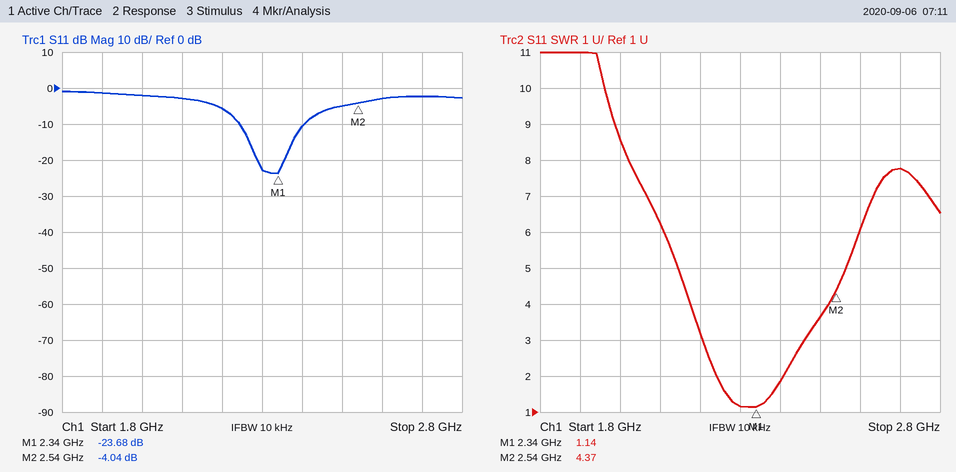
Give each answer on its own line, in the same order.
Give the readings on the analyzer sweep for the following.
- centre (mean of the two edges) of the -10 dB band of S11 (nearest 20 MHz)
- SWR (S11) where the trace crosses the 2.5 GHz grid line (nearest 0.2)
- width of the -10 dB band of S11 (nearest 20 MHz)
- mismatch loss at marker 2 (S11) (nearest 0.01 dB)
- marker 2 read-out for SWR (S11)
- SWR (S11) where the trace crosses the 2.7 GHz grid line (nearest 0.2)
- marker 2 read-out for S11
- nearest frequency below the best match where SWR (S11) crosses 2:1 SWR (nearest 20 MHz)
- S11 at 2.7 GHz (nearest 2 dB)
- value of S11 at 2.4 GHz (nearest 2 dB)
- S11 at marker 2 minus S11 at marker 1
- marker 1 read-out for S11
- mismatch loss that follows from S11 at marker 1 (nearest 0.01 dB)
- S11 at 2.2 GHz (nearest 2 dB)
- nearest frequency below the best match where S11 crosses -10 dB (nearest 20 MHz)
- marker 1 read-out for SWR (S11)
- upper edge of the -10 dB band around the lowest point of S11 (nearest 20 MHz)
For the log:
2.32 GHz
3.6
160 MHz
2.18 dB
4.37
7.8
-4.04 dB
2.24 GHz
-2 dB
-10 dB
19.64 dB
-23.68 dB
0.02 dB
-6 dB
2.24 GHz
1.14
2.40 GHz
